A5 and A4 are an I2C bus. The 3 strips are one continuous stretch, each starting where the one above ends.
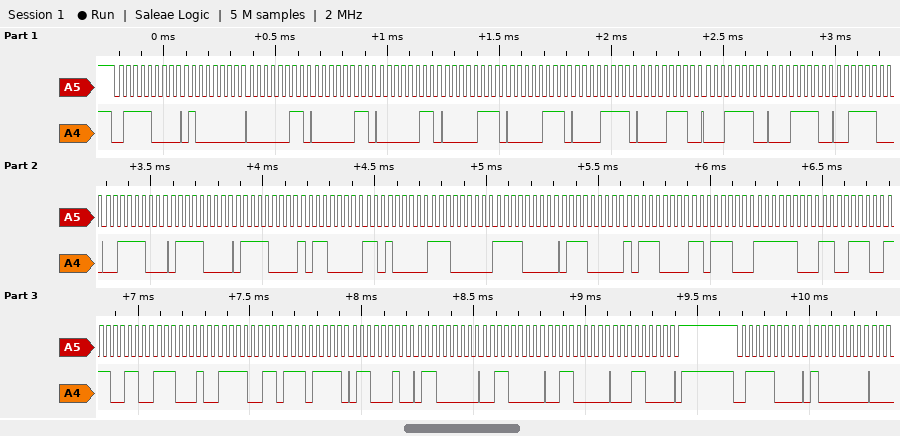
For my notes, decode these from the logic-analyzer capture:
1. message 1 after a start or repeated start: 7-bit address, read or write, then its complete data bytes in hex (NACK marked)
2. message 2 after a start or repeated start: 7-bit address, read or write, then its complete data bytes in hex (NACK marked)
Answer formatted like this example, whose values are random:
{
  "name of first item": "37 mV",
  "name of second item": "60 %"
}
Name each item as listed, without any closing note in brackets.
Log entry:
{
  "message 1 after a start or repeated start: 7-bit address, read or write, then its complete data bytes in hex": "0x3C write: 40 03 03 03 07 07 0F 0E 1E 1E 3C 3C 78 78 B0 D0 E0 F0 70 B8 DC FC CE E6 E2 F3 EF 62 60 30 30 18",
  "message 2 after a start or repeated start: 7-bit address, read or write, then its complete data bytes in hex": "0x3C write: 40"
}
